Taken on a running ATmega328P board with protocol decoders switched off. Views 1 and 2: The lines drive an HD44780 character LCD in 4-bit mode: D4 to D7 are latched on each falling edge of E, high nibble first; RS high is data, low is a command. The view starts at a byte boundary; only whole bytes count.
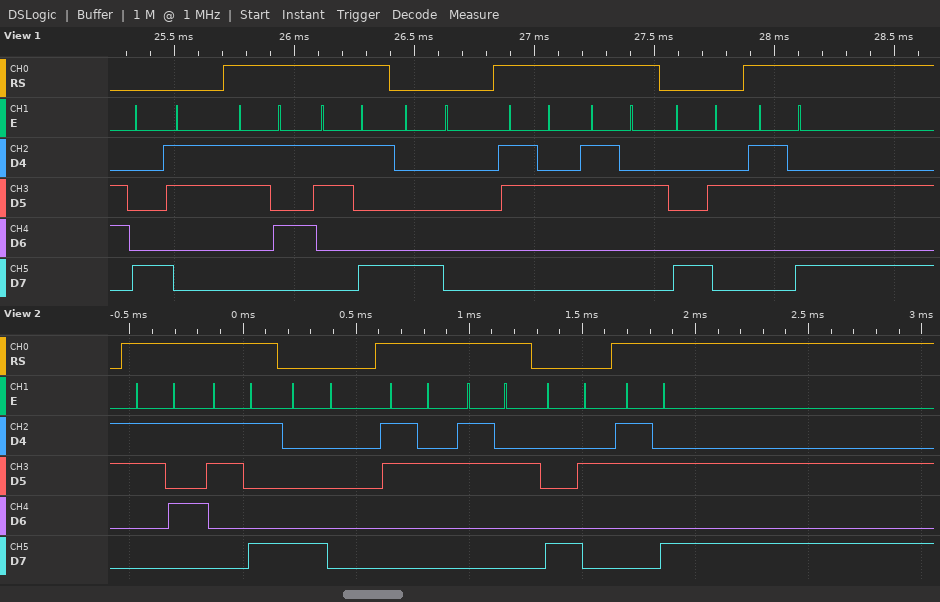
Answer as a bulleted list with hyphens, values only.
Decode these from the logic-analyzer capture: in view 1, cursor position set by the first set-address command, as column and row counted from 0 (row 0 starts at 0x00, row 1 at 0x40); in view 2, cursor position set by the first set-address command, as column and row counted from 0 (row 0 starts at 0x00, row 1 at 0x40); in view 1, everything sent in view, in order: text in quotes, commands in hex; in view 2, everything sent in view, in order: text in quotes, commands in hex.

- column 3, row 0
- column 0, row 0
- 0x83 "59" 0x80 "22" 0x82 ":"
- "59" 0x80 "22" 0x82 ":"
